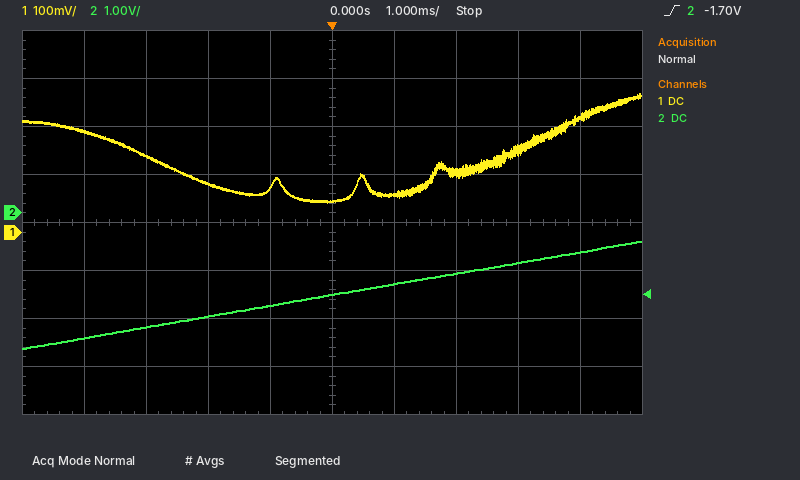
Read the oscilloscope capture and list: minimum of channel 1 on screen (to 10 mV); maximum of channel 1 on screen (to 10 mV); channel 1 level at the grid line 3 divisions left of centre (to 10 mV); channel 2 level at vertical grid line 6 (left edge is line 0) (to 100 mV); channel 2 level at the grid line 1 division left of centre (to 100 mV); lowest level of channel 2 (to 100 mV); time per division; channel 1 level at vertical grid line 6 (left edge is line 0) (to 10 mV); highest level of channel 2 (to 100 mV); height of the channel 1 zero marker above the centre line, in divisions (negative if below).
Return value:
60 mV
290 mV
160 mV
-1.5 V
-1.9 V
-2.8 V
1 ms
80 mV
-600 mV
-0.2 div
